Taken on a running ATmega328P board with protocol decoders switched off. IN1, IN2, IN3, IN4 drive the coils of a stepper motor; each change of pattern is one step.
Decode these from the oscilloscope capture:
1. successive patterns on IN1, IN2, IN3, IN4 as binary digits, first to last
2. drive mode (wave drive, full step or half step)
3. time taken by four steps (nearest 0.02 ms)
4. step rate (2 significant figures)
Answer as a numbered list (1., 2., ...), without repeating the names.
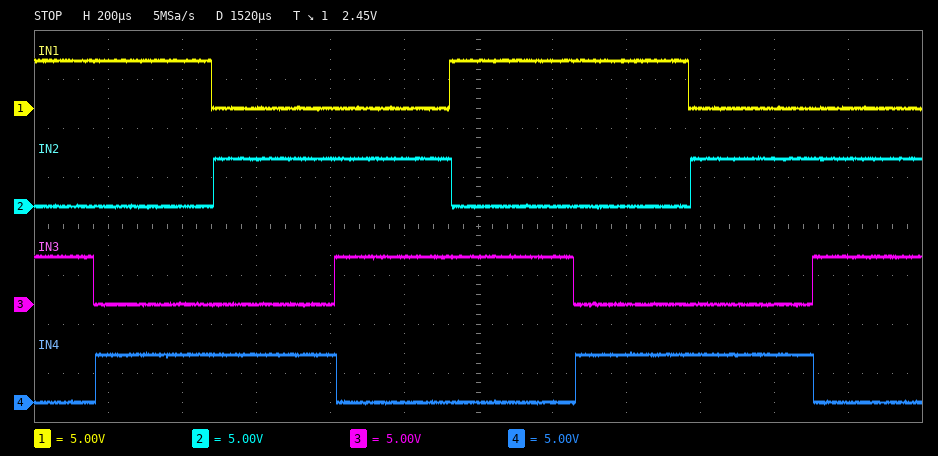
1. 1010 1001 0101 0110 1010 1001 0101 0110
2. full step
3. 1.30 ms
4. 3100 steps/s
